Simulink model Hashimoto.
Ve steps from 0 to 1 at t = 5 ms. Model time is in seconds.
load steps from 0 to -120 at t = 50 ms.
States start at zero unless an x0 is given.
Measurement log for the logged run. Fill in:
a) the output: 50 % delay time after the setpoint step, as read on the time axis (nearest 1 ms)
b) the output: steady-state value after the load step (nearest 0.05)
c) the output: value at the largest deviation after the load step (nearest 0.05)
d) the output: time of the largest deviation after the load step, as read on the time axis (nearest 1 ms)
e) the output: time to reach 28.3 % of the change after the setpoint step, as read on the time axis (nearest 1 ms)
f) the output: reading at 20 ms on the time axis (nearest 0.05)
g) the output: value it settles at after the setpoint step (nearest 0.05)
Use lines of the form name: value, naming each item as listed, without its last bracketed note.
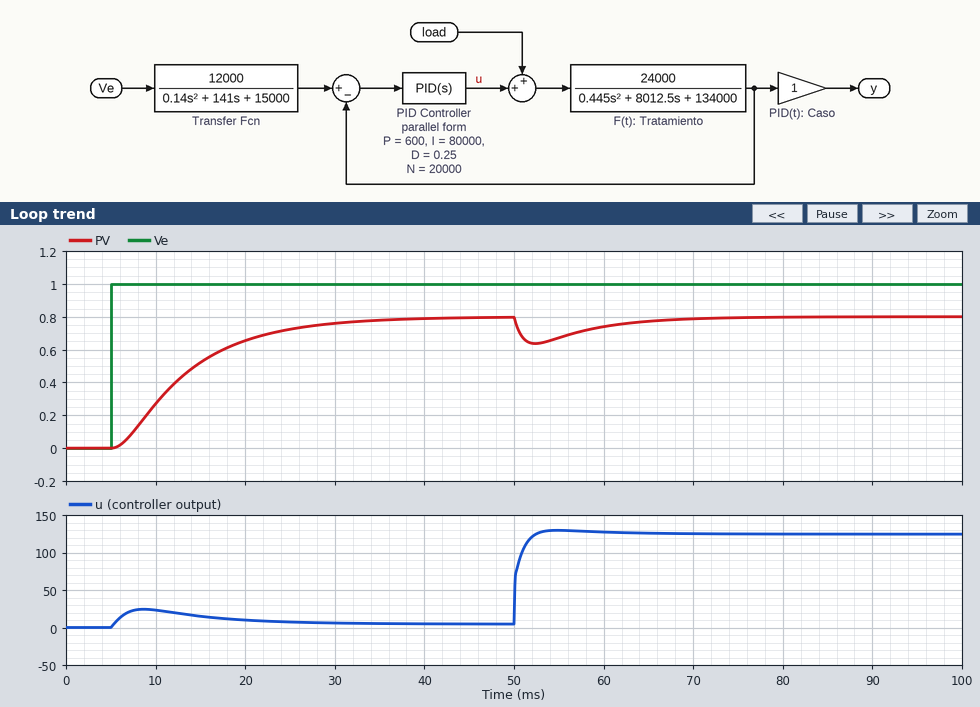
the output: 50 % delay time after the setpoint step, as read on the time axis: 12 ms
the output: steady-state value after the load step: 0.80
the output: value at the largest deviation after the load step: 0.65
the output: time of the largest deviation after the load step, as read on the time axis: 52 ms
the output: time to reach 28.3 % of the change after the setpoint step, as read on the time axis: 9 ms
the output: reading at 20 ms on the time axis: 0.65
the output: value it settles at after the setpoint step: 0.80
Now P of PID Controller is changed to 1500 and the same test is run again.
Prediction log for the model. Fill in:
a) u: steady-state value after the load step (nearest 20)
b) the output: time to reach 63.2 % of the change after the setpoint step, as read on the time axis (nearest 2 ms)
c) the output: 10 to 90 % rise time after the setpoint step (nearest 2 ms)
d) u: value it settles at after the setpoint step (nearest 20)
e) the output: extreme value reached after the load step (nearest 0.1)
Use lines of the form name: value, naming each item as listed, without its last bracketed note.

u: steady-state value after the load step: 120
the output: time to reach 63.2 % of the change after the setpoint step, as read on the time axis: 14 ms
the output: 10 to 90 % rise time after the setpoint step: 18 ms
u: value it settles at after the setpoint step: 0
the output: extreme value reached after the load step: 0.7
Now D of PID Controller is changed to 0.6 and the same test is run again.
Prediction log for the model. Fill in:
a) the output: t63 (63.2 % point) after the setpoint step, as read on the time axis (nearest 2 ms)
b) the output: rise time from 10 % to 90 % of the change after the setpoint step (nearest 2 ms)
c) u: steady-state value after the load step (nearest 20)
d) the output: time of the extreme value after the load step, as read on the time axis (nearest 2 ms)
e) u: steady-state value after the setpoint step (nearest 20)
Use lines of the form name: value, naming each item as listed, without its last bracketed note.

the output: t63 (63.2 % point) after the setpoint step, as read on the time axis: 14 ms
the output: rise time from 10 % to 90 % of the change after the setpoint step: 18 ms
u: steady-state value after the load step: 120
the output: time of the extreme value after the load step, as read on the time axis: 54 ms
u: steady-state value after the setpoint step: 0
